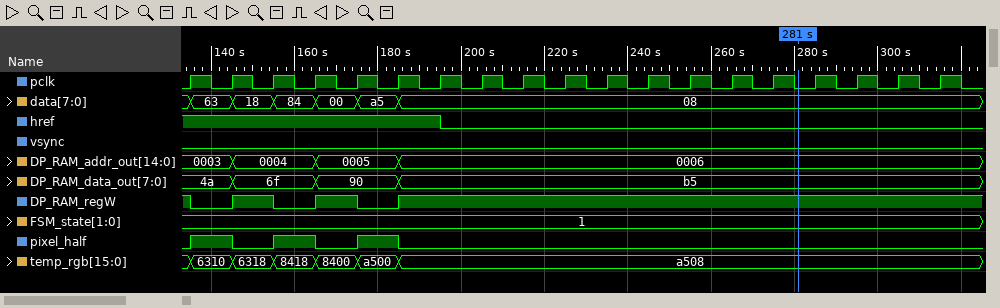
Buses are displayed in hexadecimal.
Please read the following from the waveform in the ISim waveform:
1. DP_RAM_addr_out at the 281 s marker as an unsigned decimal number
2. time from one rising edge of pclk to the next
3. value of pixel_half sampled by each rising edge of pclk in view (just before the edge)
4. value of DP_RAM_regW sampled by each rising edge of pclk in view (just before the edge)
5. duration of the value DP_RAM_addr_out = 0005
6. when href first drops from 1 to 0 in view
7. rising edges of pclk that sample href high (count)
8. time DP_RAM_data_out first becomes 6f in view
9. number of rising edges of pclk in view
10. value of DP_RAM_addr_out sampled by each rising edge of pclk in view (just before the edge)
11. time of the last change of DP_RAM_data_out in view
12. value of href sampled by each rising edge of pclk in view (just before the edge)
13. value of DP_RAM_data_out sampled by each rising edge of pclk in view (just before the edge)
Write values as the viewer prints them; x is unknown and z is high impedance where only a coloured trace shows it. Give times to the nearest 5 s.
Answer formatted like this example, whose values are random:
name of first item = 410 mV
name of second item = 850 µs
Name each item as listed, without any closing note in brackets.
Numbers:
DP_RAM_addr_out at the 281 s marker as an unsigned decimal number = 6
time from one rising edge of pclk to the next = 10 s
value of pixel_half sampled by each rising edge of pclk in view = 0 1 0 1 0 1 0 0 0 0 0 0 0 0 0 0 0 0 0
value of DP_RAM_regW sampled by each rising edge of pclk in view = 1 0 1 0 1 0 1 1 1 1 1 1 1 1 1 1 1 1 1
duration of the value DP_RAM_addr_out = 0005 = 20 s
when href first drops from 1 to 0 in view = 195 s
rising edges of pclk that sample href high = 7
time DP_RAM_data_out first becomes 6f in view = 145 s
number of rising edges of pclk in view = 19
value of DP_RAM_addr_out sampled by each rising edge of pclk in view = 0003, 0003, 0004, 0004, 0005, 0005, 0006, 0006, 0006, 0006, 0006, 0006, 0006, 0006, 0006, 0006, 0006, 0006, 0006
time of the last change of DP_RAM_data_out in view = 185 s
value of href sampled by each rising edge of pclk in view = 1 1 1 1 1 1 1 0 0 0 0 0 0 0 0 0 0 0 0
value of DP_RAM_data_out sampled by each rising edge of pclk in view = 4a, 4a, 6f, 6f, 90, 90, b5, b5, b5, b5, b5, b5, b5, b5, b5, b5, b5, b5, b5
